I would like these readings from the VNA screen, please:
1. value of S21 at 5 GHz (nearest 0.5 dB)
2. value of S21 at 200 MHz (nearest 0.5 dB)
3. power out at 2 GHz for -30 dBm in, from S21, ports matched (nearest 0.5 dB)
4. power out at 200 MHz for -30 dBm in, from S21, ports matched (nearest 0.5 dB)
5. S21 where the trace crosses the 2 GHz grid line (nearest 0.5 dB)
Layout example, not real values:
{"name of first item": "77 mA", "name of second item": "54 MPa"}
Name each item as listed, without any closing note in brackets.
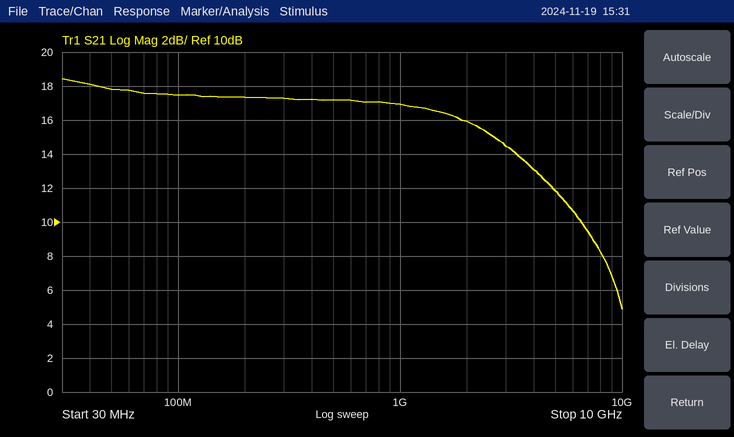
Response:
{"value of S21 at 5 GHz": "12.0 dB", "value of S21 at 200 MHz": "17.5 dB", "power out at 2 GHz for -30 dBm in, from S21, ports matched": "-14.0 dBm", "power out at 200 MHz for -30 dBm in, from S21, ports matched": "-12.5 dBm", "S21 where the trace crosses the 2 GHz grid line": "16.0 dB"}
